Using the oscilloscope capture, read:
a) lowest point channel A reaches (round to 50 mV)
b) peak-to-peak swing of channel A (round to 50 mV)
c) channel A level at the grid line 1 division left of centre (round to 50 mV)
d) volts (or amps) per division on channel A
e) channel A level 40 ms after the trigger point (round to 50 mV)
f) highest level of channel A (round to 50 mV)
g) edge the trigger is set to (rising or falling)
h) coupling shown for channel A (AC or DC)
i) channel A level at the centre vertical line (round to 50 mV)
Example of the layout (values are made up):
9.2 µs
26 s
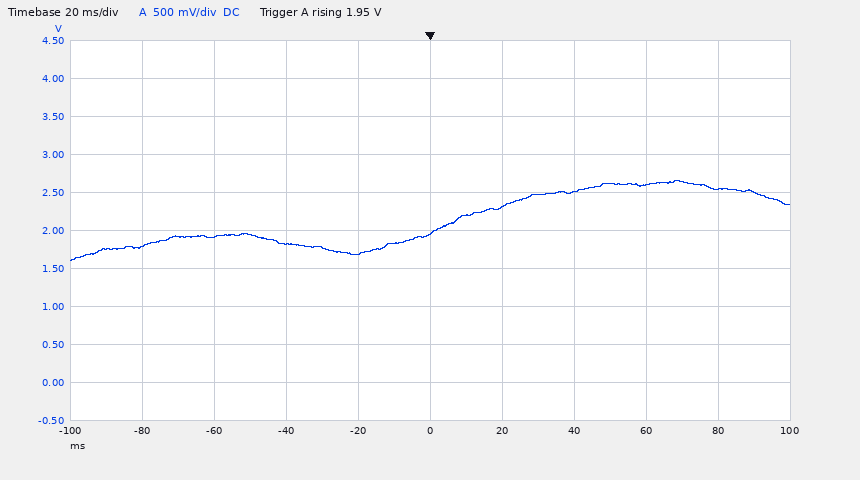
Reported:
1.60 V
1.05 V
1.70 V
500 mV
2.50 V
2.65 V
rising
DC
1.95 V
